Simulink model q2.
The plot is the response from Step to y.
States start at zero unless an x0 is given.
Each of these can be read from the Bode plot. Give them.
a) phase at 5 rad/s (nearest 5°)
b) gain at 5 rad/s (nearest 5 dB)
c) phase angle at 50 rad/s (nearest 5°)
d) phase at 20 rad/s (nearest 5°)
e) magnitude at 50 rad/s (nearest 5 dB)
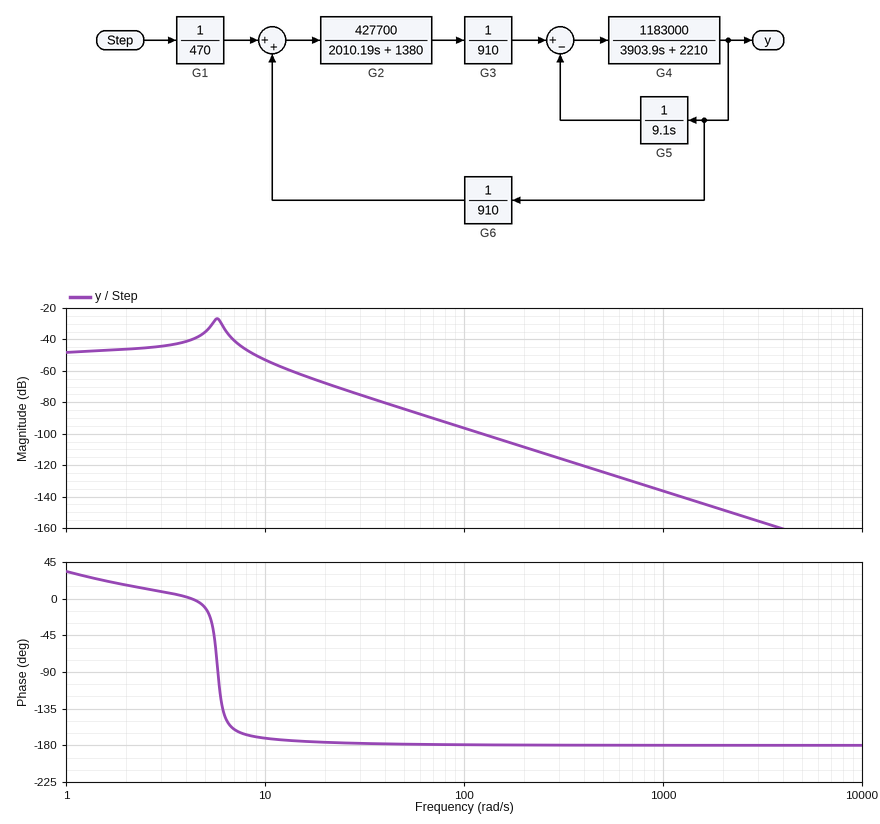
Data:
-10°
-35 dB
-180°
-175°
-85 dB
